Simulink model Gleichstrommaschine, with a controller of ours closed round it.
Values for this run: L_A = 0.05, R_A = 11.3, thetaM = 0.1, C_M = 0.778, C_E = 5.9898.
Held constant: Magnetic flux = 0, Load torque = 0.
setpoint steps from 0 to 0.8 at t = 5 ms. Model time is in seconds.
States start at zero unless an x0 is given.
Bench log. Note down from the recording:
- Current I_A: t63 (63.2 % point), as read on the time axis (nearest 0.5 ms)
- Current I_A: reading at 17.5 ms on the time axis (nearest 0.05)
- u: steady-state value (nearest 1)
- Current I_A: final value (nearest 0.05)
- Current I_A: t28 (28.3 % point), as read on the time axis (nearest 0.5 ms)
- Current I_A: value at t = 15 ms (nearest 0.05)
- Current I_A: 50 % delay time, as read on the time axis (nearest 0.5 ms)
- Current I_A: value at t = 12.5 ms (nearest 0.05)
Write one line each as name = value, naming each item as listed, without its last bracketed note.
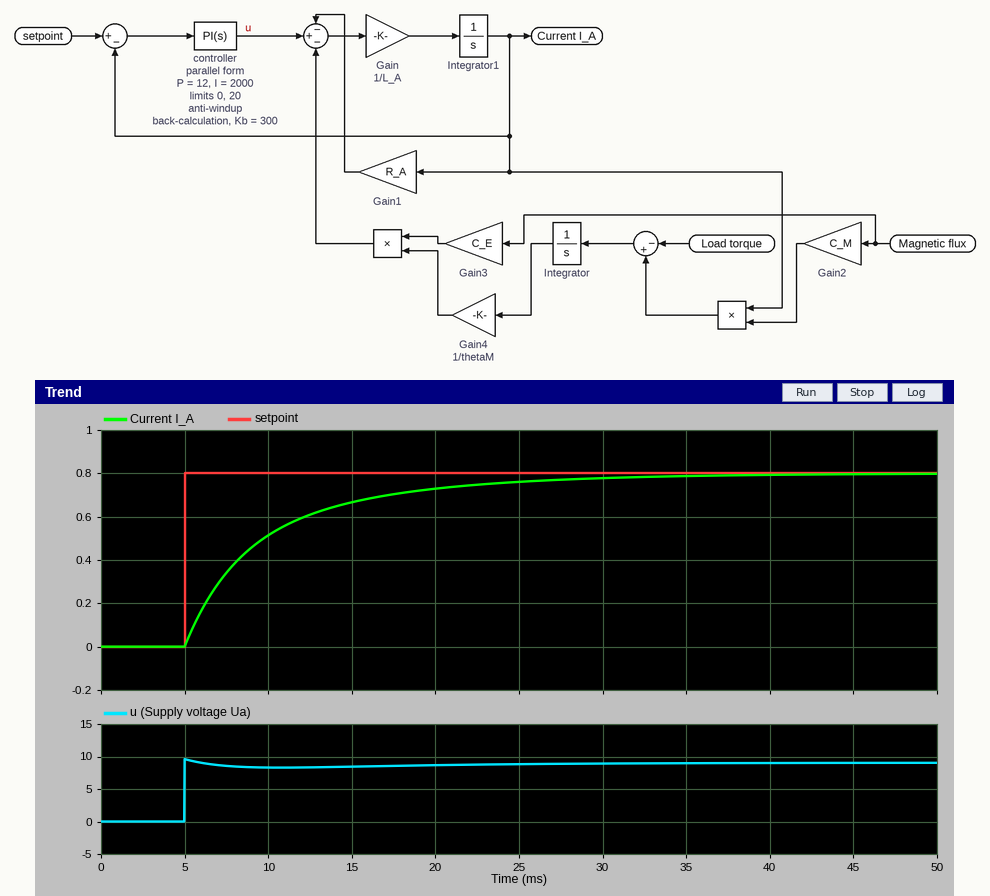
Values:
Current I_A: t63 (63.2 % point), as read on the time axis = 10.0 ms
Current I_A: reading at 17.5 ms on the time axis = 0.70
u: steady-state value = 9
Current I_A: final value = 0.80
Current I_A: t28 (28.3 % point), as read on the time axis = 6.5 ms
Current I_A: value at t = 15 ms = 0.65
Current I_A: 50 % delay time, as read on the time axis = 8.0 ms
Current I_A: value at t = 12.5 ms = 0.60
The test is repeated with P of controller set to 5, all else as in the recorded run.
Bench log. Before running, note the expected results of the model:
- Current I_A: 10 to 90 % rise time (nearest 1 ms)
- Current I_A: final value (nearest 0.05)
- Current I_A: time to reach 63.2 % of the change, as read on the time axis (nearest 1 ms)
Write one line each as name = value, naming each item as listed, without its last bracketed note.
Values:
Current I_A: 10 to 90 % rise time = 11 ms
Current I_A: final value = 0.80
Current I_A: time to reach 63.2 % of the change, as read on the time axis = 12 ms
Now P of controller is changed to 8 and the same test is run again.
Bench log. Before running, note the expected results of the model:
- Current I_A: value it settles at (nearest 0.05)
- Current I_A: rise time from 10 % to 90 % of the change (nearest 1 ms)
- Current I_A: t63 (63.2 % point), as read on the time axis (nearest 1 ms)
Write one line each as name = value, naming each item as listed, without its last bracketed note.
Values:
Current I_A: value it settles at = 0.80
Current I_A: rise time from 10 % to 90 % of the change = 12 ms
Current I_A: t63 (63.2 % point), as read on the time axis = 11 ms
